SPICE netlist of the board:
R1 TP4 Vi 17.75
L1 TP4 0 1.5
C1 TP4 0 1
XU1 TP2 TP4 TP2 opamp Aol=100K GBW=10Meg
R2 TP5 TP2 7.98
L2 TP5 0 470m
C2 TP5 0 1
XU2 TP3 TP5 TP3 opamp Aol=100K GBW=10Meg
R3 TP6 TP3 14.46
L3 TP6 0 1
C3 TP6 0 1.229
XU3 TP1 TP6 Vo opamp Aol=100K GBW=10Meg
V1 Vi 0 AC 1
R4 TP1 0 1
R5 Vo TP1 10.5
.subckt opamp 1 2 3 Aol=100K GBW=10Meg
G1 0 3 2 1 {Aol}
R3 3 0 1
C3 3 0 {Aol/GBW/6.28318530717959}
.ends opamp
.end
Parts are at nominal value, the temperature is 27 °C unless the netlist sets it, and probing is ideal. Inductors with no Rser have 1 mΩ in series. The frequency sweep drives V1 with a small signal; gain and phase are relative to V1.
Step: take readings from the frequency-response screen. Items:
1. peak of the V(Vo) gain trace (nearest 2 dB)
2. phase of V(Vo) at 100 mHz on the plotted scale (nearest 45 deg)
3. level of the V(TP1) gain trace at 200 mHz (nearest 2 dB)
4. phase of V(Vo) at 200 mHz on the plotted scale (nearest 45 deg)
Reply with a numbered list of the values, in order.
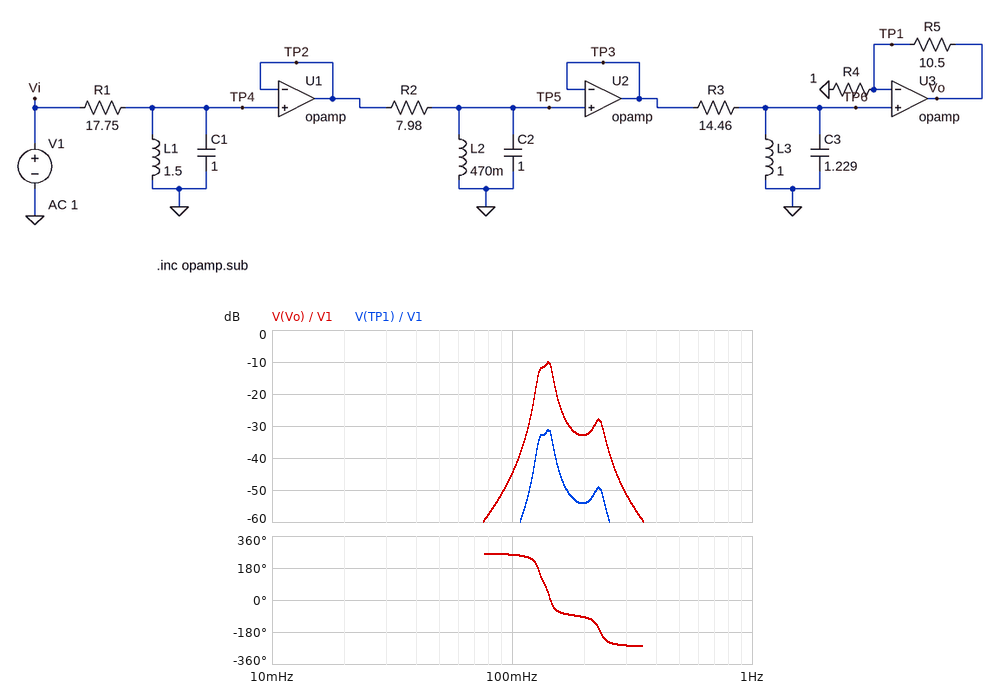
1. -10 dB
2. 270 deg
3. -54 dB
4. -90 deg
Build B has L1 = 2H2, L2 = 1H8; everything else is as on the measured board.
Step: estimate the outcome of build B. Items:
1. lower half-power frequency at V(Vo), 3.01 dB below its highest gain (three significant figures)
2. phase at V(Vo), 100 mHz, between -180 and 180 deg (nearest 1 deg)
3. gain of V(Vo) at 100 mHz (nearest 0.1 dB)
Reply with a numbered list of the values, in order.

1. 105 mHz
2. -152 deg
3. -13.3 dB
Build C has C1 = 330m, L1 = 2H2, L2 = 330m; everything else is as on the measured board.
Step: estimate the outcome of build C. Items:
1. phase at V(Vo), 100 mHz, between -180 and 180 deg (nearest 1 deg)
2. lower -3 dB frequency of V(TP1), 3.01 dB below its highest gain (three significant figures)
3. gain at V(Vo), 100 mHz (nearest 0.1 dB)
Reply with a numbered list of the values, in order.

1. -103 deg
2. 140 mHz
3. -50.1 dB
